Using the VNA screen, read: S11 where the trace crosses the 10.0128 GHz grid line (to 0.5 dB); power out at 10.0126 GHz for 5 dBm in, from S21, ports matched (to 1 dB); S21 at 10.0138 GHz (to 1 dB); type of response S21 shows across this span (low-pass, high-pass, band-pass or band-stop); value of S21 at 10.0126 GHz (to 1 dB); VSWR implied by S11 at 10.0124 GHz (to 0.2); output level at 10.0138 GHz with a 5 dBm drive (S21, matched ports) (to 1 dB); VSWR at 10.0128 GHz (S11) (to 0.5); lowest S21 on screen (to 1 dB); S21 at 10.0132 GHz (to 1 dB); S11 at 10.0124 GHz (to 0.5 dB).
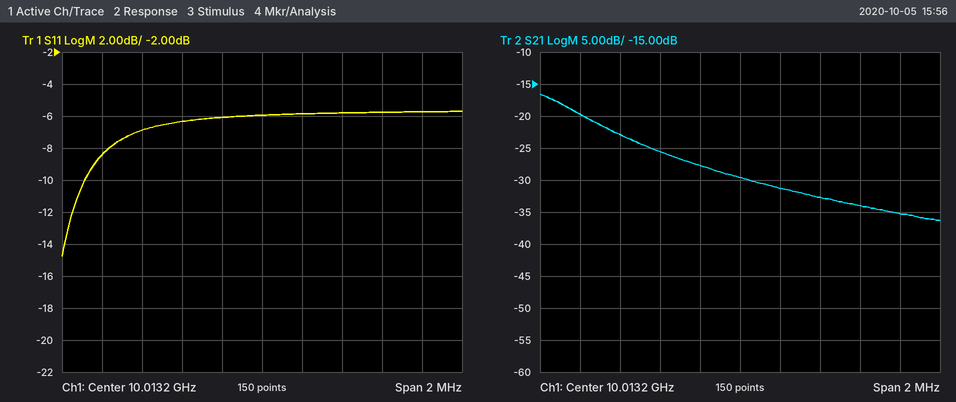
-6.5 dB
-18 dBm
-34 dB
low-pass
-23 dB
2.2
-29 dBm
3.0
-36 dB
-30 dB
-8.5 dB
